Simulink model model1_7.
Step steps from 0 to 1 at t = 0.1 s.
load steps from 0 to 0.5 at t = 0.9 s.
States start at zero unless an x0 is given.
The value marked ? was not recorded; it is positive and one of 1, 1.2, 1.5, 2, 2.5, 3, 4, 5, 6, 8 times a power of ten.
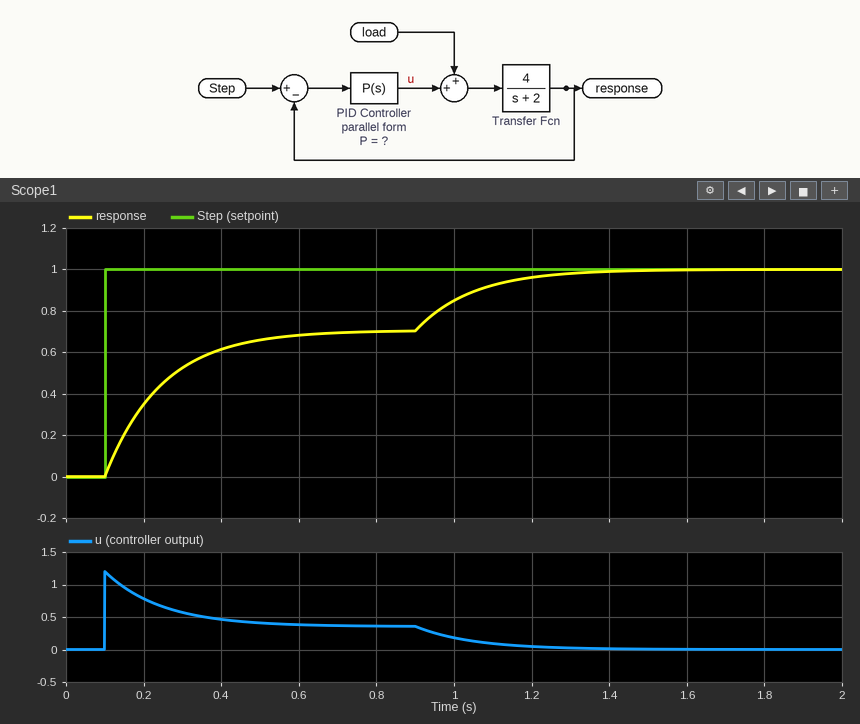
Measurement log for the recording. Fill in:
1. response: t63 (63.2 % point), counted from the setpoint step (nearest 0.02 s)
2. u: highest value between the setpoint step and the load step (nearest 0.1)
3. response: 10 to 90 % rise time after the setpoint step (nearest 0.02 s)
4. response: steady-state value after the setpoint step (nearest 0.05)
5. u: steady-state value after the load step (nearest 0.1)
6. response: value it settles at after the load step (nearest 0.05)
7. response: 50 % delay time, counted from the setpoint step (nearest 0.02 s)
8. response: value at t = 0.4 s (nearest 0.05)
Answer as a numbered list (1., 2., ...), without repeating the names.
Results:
1. 0.14 s
2. 1.2
3. 0.32 s
4. 0.70
5. 0.0
6. 1.00
7. 0.10 s
8. 0.60
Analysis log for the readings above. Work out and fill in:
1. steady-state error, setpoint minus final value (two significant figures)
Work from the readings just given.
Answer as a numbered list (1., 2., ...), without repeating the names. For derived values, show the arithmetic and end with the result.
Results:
1. 1 - 0.7 = 0.30
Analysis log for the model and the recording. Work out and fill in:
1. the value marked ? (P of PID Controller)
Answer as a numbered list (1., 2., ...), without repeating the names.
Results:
1. 1.2
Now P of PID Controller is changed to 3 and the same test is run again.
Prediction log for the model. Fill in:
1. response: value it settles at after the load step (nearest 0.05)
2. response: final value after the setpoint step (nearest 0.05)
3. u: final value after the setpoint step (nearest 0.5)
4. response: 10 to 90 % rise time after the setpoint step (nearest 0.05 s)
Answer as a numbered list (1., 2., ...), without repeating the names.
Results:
1. 1.00
2. 0.85
3. 0.5
4. 0.15 s
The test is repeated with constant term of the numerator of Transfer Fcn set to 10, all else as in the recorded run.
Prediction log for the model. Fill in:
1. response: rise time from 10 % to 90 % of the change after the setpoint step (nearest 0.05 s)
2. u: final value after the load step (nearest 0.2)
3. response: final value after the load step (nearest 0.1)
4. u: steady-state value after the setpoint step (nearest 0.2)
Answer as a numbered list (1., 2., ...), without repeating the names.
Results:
1. 0.15 s
2. -0.2
3. 1.2
4. 0.2
